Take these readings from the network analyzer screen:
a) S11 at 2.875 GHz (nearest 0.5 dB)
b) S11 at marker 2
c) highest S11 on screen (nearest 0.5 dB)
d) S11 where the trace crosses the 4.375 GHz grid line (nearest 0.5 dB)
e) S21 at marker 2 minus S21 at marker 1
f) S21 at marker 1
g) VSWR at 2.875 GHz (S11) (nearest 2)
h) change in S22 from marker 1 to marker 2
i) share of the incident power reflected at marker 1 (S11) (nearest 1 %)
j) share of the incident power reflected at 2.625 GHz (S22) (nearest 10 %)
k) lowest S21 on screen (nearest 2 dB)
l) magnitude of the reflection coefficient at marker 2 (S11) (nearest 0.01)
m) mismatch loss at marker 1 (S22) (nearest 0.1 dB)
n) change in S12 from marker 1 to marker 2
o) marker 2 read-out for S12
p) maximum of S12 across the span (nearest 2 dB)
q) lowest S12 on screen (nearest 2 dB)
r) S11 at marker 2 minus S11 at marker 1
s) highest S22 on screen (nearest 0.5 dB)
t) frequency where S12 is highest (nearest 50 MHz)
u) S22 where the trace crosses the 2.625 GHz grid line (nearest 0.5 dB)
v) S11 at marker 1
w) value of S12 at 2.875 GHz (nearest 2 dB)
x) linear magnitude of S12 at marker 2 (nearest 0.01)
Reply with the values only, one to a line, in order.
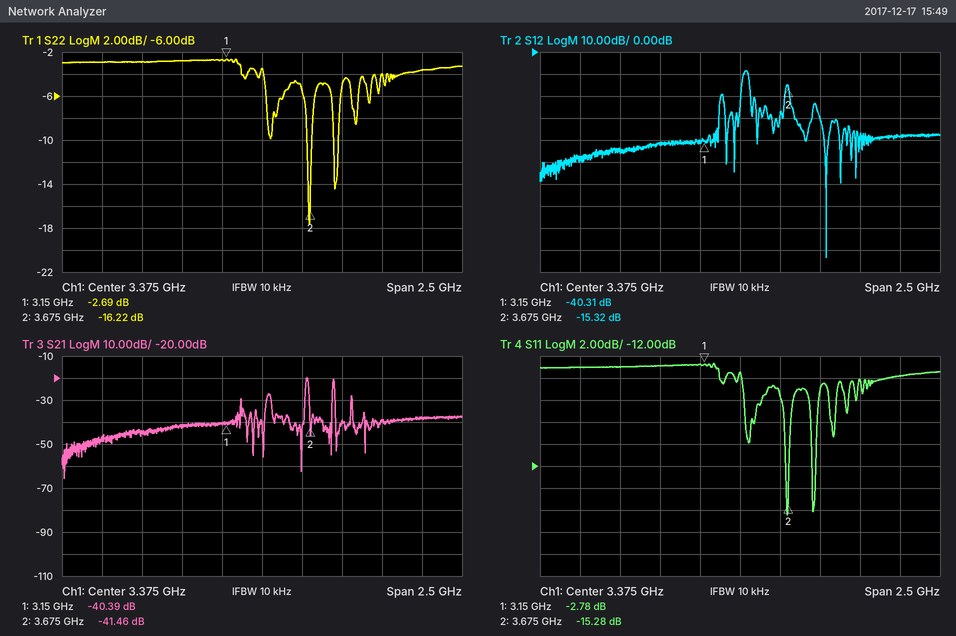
-3.0 dB
-15.28 dB
-2.5 dB
-4.0 dB
-1.07 dB
-40.39 dB
6
-13.53 dB
53 %
50 %
-66 dB
0.17
3.4 dB
24.99 dB
-15.32 dB
-8 dB
-94 dB
-12.50 dB
-2.5 dB
3.40 GHz
-3.0 dB
-2.78 dB
-42 dB
0.17
